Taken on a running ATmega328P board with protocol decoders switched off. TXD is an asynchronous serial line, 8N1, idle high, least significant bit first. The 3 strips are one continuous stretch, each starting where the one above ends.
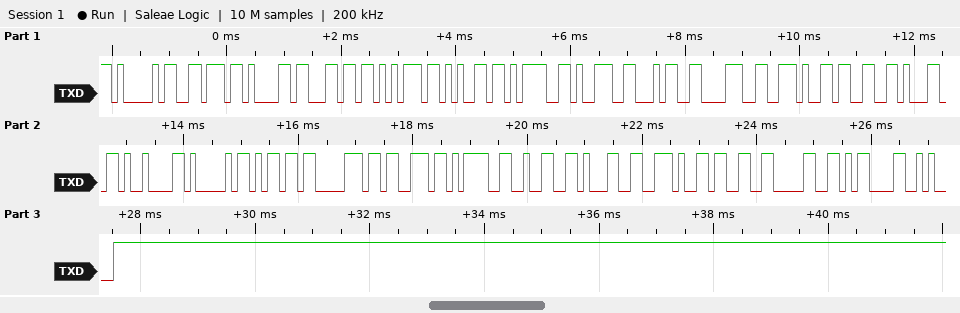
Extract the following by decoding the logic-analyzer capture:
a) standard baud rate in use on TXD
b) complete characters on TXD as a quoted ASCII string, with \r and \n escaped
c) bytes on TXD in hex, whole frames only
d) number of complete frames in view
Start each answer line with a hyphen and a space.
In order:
- 9600 baud
- "Avalue=948.31\tAmps=21.30\r\n"
- 41 76 61 6C 75 65 3D 39 34 38 2E 33 31 09 41 6D 70 73 3D 32 31 2E 33 30 0D 0A
- 26
